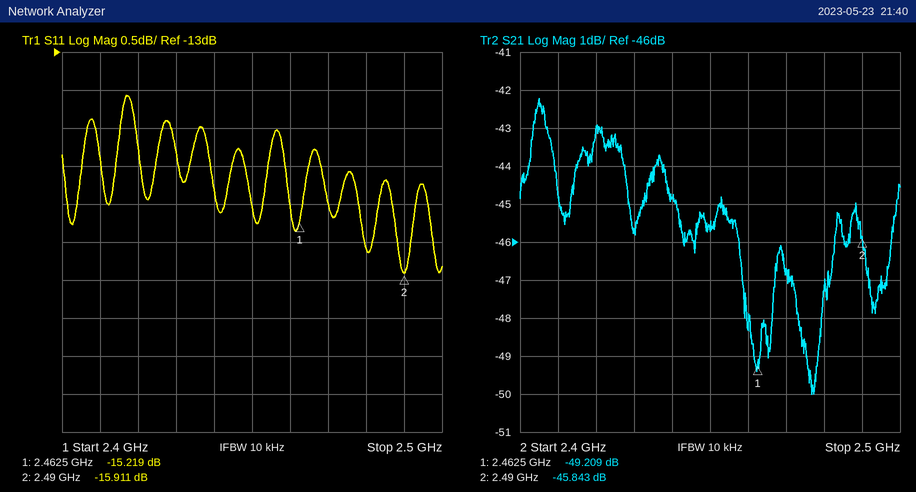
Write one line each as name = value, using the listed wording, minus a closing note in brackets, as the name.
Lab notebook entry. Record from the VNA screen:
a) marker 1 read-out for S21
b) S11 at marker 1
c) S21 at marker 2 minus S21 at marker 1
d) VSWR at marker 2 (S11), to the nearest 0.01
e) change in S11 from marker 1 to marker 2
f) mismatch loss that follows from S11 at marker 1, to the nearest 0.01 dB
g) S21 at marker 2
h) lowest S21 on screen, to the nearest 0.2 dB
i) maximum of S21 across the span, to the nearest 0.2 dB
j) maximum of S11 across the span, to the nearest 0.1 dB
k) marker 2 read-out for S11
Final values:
marker 1 read-out for S21 = -49.209 dB
S11 at marker 1 = -15.219 dB
S21 at marker 2 minus S21 at marker 1 = 3.366 dB
VSWR at marker 2 (S11), to the nearest 0.01 = 1.38
change in S11 from marker 1 to marker 2 = -0.692 dB
mismatch loss that follows from S11 at marker 1, to the nearest 0.01 dB = 0.13 dB
S21 at marker 2 = -45.843 dB
lowest S21 on screen, to the nearest 0.2 dB = -50.0 dB
maximum of S21 across the span, to the nearest 0.2 dB = -42.2 dB
maximum of S11 across the span, to the nearest 0.1 dB = -13.6 dB
marker 2 read-out for S11 = -15.911 dB
